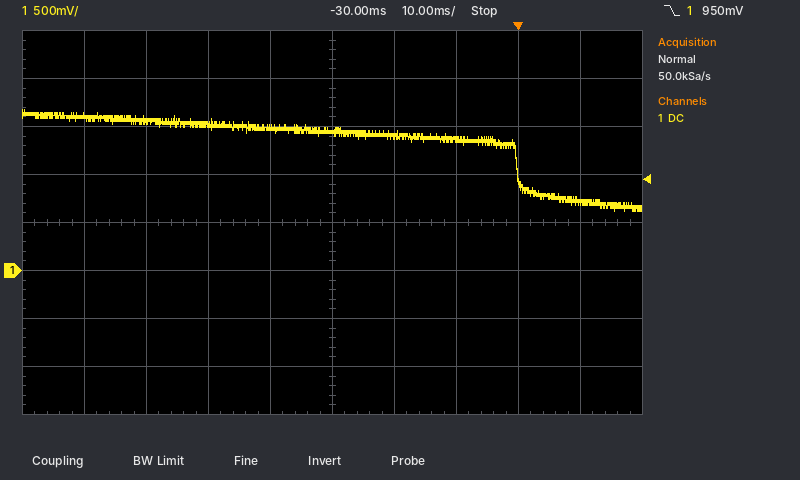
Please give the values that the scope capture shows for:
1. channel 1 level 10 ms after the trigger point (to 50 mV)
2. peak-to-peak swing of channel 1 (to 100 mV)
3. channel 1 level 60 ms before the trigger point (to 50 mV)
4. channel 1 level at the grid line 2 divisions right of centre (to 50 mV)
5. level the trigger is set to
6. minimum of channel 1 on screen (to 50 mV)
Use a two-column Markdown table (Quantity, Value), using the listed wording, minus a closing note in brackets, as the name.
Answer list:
| Quantity | Value |
|---|---|
| channel 1 level 10 ms after the trigger point | 700 mV |
| peak-to-peak swing of channel 1 | 1.10 V |
| channel 1 level 60 ms before the trigger point | 1.55 V |
| channel 1 level at the grid line 2 divisions right of centre | 1.35 V |
| level the trigger is set to | 950 mV |
| minimum of channel 1 on screen | 600 mV |
